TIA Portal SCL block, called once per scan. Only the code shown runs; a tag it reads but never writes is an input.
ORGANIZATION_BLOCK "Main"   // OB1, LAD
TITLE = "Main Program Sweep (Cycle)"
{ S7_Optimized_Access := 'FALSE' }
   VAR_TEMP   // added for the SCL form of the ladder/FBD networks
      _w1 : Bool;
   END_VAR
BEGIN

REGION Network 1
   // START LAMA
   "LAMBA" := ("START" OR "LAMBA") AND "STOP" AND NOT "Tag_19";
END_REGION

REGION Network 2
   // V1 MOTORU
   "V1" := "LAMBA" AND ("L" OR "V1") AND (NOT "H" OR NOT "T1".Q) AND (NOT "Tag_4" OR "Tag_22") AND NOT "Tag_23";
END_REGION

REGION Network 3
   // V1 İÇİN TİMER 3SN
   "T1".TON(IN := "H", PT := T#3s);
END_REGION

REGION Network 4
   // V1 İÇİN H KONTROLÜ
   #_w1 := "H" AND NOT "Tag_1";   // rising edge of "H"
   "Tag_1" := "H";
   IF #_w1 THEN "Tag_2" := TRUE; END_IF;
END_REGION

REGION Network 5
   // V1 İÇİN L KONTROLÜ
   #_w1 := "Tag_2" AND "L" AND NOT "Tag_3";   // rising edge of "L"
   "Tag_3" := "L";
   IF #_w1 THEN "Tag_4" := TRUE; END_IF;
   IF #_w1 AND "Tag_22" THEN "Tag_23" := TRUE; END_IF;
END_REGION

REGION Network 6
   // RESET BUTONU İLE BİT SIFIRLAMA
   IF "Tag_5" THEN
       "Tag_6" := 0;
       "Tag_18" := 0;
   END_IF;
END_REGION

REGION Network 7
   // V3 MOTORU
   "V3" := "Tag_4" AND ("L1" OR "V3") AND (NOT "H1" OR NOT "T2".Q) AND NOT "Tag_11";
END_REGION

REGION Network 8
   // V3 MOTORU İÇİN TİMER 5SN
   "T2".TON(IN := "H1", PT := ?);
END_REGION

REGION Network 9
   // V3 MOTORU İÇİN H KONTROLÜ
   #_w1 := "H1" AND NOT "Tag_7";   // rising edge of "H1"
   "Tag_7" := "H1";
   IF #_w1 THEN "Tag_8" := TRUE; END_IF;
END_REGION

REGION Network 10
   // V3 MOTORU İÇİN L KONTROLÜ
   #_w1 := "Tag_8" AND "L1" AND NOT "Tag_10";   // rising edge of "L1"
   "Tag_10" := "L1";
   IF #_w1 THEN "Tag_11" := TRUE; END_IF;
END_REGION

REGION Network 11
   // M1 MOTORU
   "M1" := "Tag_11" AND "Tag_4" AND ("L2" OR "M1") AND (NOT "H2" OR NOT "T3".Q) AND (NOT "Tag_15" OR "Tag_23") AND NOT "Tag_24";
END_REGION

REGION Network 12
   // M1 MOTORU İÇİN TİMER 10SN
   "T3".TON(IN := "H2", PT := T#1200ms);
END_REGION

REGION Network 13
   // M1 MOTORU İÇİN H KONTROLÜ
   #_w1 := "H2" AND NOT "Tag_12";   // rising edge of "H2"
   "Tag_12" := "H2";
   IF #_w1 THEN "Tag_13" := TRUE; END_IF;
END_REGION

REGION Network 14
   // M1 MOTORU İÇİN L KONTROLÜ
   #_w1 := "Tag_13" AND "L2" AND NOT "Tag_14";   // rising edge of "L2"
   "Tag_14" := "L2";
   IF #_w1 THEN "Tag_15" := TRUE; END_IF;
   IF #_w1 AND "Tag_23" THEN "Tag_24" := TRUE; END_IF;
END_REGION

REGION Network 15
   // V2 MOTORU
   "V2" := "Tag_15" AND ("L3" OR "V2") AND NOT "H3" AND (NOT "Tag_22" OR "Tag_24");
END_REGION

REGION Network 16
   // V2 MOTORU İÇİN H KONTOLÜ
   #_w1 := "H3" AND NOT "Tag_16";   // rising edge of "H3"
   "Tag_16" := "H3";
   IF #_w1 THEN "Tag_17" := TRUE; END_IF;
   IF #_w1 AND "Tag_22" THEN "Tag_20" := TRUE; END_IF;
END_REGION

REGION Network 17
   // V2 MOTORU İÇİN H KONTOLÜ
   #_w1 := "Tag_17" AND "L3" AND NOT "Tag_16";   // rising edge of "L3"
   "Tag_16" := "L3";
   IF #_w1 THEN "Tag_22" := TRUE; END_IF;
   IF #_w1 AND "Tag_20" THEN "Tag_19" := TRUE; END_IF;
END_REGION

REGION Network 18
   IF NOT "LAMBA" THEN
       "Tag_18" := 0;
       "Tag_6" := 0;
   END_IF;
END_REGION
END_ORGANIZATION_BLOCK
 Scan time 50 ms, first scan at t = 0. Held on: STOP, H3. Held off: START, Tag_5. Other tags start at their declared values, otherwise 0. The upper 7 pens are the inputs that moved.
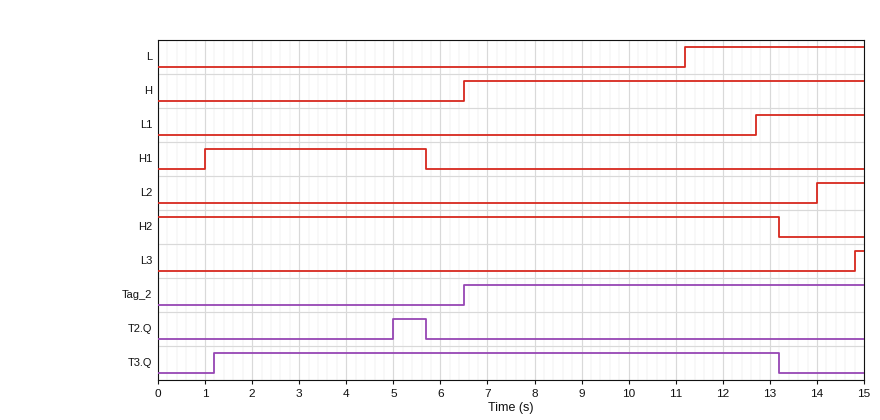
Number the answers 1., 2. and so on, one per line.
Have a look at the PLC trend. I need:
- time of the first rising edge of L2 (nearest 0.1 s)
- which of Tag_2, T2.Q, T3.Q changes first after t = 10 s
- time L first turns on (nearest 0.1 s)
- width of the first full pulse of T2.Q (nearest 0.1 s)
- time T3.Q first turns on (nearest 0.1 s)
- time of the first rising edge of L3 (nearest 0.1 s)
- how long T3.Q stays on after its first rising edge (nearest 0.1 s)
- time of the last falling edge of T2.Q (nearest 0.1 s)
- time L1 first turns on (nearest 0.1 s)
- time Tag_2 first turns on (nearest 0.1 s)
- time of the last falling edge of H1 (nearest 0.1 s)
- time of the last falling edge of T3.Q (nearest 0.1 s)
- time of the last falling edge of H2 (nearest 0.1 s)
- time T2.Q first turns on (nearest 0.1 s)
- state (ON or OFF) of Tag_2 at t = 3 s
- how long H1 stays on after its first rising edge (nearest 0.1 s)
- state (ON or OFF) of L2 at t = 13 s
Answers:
1. 14.0 s
2. T3.Q
3. 11.2 s
4. 0.7 s
5. 1.2 s
6. 14.8 s
7. 12.0 s
8. 5.7 s
9. 12.7 s
10. 6.5 s
11. 5.7 s
12. 13.2 s
13. 13.2 s
14. 5.0 s
15. OFF
16. 4.7 s
17. OFF
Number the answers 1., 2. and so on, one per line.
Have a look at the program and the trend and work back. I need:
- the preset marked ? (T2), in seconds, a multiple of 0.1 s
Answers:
1. 4.0 s
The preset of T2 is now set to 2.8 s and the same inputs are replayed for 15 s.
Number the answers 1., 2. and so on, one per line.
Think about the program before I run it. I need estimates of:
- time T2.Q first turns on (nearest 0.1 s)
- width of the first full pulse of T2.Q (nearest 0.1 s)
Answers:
1. 3.8 s
2. 1.9 s
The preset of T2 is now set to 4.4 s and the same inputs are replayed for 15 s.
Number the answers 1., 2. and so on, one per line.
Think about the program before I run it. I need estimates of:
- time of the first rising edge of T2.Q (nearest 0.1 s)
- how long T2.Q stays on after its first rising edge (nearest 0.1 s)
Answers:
1. 5.4 s
2. 0.3 s
